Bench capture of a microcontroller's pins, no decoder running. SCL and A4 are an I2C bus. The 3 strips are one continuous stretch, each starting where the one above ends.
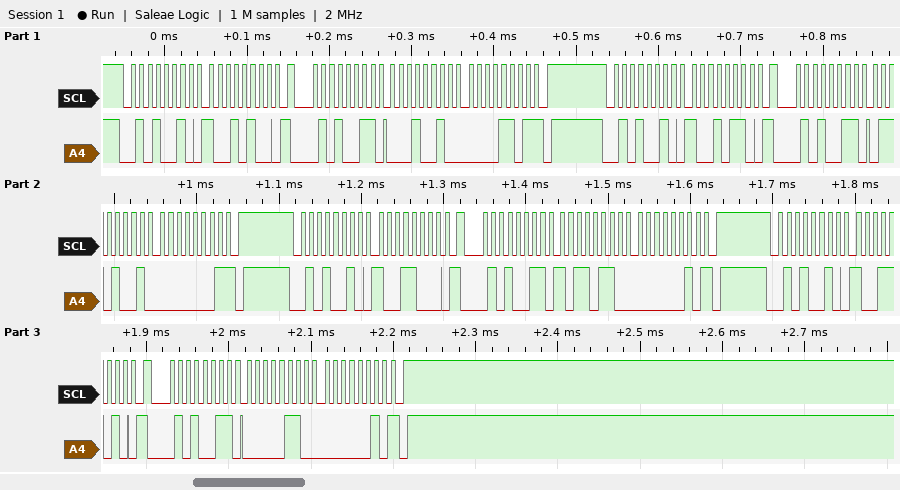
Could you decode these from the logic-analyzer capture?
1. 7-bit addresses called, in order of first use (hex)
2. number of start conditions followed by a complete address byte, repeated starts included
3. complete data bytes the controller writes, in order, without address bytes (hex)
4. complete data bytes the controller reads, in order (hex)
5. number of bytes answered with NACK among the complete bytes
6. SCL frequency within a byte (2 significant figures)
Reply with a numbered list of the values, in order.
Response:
1. 0x29
2. 8
3. 94 96 98 9A
4. 12 0D 69 01 B6 02 06 02
5. 4
6. 100 kHz
